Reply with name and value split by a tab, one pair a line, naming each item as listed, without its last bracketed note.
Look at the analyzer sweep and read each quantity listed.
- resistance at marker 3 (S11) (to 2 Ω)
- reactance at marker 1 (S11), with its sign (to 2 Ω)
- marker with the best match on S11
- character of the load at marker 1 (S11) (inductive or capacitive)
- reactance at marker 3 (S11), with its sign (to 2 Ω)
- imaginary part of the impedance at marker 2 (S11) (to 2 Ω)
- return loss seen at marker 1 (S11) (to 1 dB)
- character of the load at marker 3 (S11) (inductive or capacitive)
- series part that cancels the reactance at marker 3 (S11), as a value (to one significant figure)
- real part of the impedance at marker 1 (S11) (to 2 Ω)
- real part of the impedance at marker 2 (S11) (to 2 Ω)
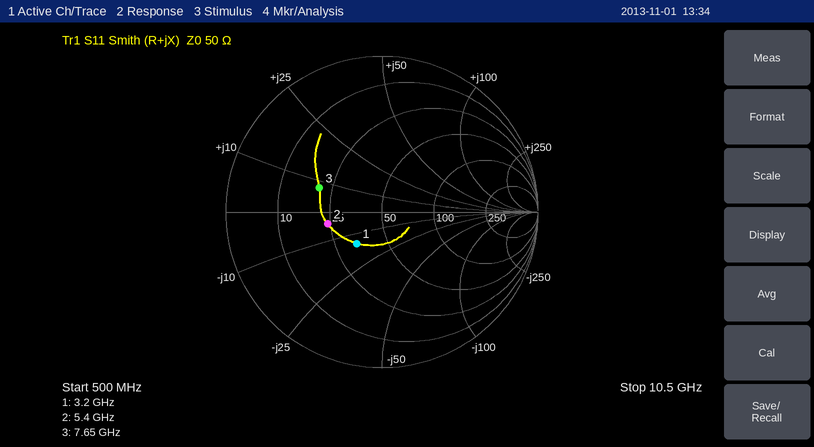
resistance at marker 3 (S11)	20 Ω
reactance at marker 1 (S11), with its sign	-14 Ω
marker with the best match on S11	marker 1
character of the load at marker 1 (S11)	capacitive
reactance at marker 3 (S11), with its sign	+8 Ω
imaginary part of the impedance at marker 2 (S11)	-4 Ω
return loss seen at marker 1 (S11)	12 dB
character of the load at marker 3 (S11)	inductive
series part that cancels the reactance at marker 3 (S11), as a value	3 pF
real part of the impedance at marker 1 (S11)	34 Ω
real part of the impedance at marker 2 (S11)	24 Ω
